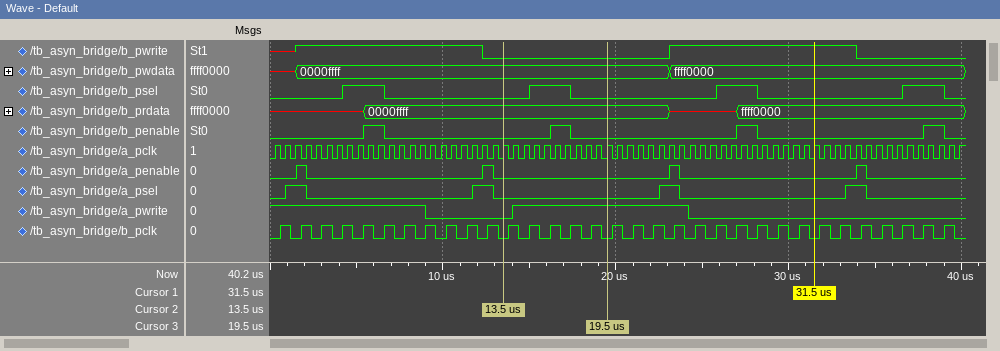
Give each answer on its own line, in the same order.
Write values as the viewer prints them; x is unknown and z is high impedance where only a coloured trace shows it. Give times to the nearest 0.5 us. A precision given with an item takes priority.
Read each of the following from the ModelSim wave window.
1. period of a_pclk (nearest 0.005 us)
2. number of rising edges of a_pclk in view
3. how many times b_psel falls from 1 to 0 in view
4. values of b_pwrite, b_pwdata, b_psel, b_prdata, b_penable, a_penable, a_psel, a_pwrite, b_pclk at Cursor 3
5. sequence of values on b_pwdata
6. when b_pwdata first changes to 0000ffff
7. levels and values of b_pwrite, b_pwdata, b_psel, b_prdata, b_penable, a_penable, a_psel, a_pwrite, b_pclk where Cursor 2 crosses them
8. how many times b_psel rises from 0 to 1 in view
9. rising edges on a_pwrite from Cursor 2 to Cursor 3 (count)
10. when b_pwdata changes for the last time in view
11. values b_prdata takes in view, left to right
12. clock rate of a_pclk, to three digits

0.6 us
67
4
b_pwrite=0, b_pwdata=0000ffff, b_psel=0, b_prdata=0000ffff, b_penable=0, a_penable=0, a_psel=0, a_pwrite=1, b_pclk=0
x, 0000ffff, ffff0000
1.5 us
b_pwrite=0, b_pwdata=0000ffff, b_psel=0, b_prdata=0000ffff, b_penable=0, a_penable=0, a_psel=0, a_pwrite=0, b_pclk=0
4
1
23 us
x, 0000ffff, x, ffff0000
1.67 MHz
